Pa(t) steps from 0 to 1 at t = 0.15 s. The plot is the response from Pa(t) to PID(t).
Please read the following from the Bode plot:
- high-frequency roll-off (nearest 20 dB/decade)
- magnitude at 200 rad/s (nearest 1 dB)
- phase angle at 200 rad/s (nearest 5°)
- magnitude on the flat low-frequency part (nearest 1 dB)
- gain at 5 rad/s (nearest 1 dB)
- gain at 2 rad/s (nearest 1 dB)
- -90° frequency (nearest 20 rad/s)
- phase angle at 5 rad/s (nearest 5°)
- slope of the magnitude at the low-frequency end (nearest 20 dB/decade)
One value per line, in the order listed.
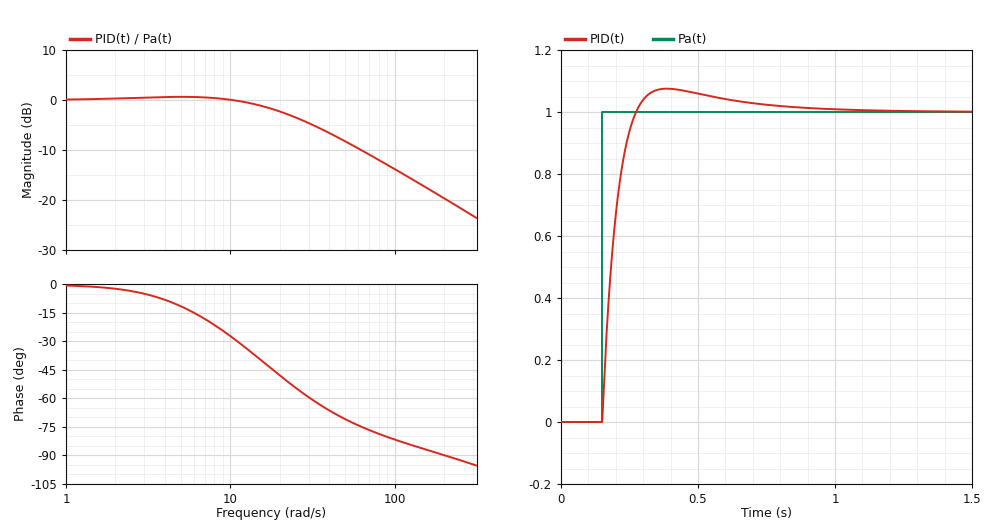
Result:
-20 dB/decade
-20 dB
-90°
0 dB
1 dB
0 dB
200 rad/s
-10°
0 dB/decade
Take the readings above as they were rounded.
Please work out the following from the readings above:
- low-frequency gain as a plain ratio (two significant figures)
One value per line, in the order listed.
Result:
1.0
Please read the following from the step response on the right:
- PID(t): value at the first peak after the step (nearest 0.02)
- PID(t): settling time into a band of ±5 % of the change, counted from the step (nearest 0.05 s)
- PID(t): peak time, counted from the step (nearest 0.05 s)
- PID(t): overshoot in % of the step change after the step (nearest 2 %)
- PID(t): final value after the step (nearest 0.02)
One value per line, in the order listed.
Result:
1.08
0.40 s
0.25 s
8 %
1.00
